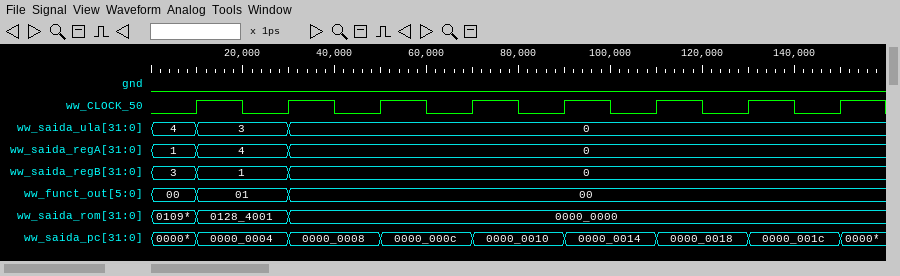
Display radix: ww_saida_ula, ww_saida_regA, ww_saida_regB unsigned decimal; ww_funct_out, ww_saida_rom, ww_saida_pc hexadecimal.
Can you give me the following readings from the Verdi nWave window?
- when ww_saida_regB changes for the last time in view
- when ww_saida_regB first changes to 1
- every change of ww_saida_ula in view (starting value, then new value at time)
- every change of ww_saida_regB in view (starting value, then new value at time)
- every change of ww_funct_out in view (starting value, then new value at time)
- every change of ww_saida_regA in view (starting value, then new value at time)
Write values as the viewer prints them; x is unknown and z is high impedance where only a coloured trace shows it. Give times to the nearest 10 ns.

30 ns
10 ns
4, 3 at 10 ns, 0 at 30 ns
3, 1 at 10 ns, 0 at 30 ns
00, 01 at 10 ns, 00 at 30 ns
1, 4 at 10 ns, 0 at 30 ns
